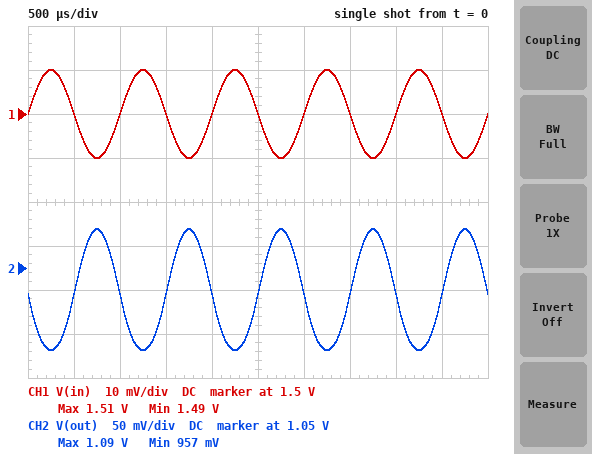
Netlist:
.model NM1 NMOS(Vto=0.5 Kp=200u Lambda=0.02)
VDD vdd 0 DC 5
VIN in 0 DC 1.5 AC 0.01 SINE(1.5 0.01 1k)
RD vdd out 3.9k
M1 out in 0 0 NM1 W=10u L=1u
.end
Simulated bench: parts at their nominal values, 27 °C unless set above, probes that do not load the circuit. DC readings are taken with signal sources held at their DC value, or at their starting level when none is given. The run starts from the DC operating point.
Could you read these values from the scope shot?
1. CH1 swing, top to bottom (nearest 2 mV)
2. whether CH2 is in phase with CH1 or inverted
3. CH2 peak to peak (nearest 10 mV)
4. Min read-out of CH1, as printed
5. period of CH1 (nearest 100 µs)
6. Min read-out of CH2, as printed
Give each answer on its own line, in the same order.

20 mV
inverted
140 mV
1.49 V
1.0 ms
957 mV
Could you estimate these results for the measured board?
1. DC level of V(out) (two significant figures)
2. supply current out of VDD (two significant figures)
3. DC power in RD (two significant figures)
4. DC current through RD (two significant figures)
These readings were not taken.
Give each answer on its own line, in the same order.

1.0 V
1.0 mA
4.1 mW
1.0 mA
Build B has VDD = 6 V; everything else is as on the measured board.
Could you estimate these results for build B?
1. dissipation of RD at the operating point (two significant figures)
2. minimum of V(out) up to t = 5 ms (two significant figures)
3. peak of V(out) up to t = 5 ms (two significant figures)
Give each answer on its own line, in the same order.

4.2 mW
1.9 V
2.0 V
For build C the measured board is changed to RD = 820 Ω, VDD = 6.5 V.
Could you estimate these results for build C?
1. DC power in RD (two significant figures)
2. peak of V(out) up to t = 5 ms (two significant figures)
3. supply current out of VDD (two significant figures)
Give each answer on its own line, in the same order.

1.0 mW
5.6 V
1.1 mA
